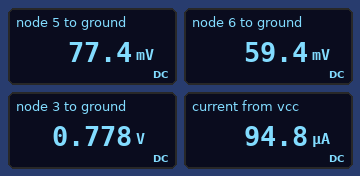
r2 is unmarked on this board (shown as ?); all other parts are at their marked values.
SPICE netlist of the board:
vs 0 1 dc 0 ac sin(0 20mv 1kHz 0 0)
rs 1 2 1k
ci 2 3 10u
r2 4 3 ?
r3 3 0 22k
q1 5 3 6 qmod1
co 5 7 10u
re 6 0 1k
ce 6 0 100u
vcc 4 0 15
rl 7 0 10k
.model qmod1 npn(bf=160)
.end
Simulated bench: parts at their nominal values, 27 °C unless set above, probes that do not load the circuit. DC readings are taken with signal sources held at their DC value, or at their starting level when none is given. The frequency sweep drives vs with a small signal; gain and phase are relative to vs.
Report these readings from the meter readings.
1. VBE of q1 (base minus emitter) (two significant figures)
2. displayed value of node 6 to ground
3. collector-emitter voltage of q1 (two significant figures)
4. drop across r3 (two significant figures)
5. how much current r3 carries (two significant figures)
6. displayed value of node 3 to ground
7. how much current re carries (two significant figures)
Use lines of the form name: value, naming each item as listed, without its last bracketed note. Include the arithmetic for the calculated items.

VBE of q1 (base minus emitter): 778 mV - 59.4 mV = 720 mV
displayed value of node 6 to ground: 59.4 mV
collector-emitter voltage of q1: 77.4 mV - 59.4 mV = 18 mV
drop across r3: 778 mV = 780 mV
how much current r3 carries: (778 mV) / 22 kΩ = 35 µA
displayed value of node 3 to ground: 0.778 V
how much current re carries: (59.4 mV) / 1 kΩ = 59 µA
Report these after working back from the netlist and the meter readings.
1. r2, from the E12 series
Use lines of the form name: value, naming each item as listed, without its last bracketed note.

r2, from the E12 series: 150 kΩ
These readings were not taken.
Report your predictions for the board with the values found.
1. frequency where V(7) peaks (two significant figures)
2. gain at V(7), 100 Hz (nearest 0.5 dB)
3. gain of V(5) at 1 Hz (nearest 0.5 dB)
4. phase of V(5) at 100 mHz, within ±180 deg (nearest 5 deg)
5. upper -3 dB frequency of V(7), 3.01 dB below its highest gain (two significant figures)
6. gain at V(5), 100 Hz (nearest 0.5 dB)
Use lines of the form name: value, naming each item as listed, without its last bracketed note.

frequency where V(7) peaks: 5.5 Hz
gain at V(7), 100 Hz: -39.5 dB
gain of V(5) at 1 Hz: -26.5 dB
phase of V(5) at 100 mHz, within ±180 deg: -95 deg
upper -3 dB frequency of V(7), 3.01 dB below its highest gain: 17 Hz
gain at V(5), 100 Hz: -39.5 dB
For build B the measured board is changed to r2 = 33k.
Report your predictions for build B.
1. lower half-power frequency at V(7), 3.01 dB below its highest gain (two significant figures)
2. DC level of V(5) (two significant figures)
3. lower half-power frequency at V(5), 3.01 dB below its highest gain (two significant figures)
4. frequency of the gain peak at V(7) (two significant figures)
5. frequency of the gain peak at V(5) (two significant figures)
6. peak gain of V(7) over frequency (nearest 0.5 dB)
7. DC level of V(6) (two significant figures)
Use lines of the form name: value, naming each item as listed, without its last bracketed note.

lower half-power frequency at V(7), 3.01 dB below its highest gain: 2.1 Hz
DC level of V(5): 390 mV
lower half-power frequency at V(5), 3.01 dB below its highest gain: 1.4 Hz
frequency of the gain peak at V(7): 6.4 Hz
frequency of the gain peak at V(5): 5.4 Hz
peak gain of V(7) over frequency: -22.0 dB
DC level of V(6): 370 mV
